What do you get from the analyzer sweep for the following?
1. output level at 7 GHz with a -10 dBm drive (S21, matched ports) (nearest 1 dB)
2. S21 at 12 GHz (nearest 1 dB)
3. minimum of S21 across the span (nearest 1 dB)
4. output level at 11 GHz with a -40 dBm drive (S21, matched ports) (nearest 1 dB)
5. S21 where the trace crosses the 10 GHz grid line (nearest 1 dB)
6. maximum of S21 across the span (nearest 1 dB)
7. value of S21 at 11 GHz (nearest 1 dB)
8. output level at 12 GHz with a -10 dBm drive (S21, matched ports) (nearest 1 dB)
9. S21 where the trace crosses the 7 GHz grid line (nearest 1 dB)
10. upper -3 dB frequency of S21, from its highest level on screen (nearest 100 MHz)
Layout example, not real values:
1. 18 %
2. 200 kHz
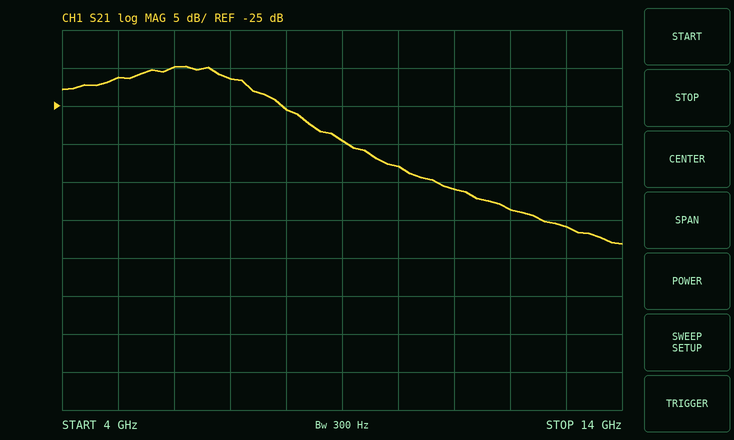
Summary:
1. -31 dBm
2. -39 dB
3. -43 dB
4. -76 dBm
5. -33 dB
6. -20 dB
7. -36 dB
8. -49 dBm
9. -21 dB
10. 7.4 GHz
